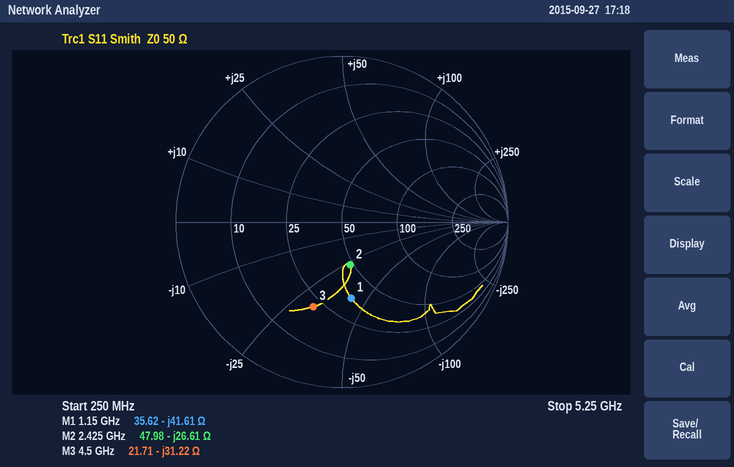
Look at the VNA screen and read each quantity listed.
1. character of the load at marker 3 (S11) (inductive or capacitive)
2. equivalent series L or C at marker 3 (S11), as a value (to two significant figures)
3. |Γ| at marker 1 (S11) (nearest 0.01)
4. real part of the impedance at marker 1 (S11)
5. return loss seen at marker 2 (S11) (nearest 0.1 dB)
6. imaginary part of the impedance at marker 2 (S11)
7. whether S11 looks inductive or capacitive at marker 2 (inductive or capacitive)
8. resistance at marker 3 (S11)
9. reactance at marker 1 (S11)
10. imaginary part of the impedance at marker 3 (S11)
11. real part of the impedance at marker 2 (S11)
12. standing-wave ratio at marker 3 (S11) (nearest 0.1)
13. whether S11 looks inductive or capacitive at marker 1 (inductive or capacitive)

capacitive
1.1 pF
0.46
35.62 Ω
11.6 dB
-26.61 Ω
capacitive
21.71 Ω
-41.61 Ω
-31.22 Ω
47.98 Ω
3.3
capacitive
